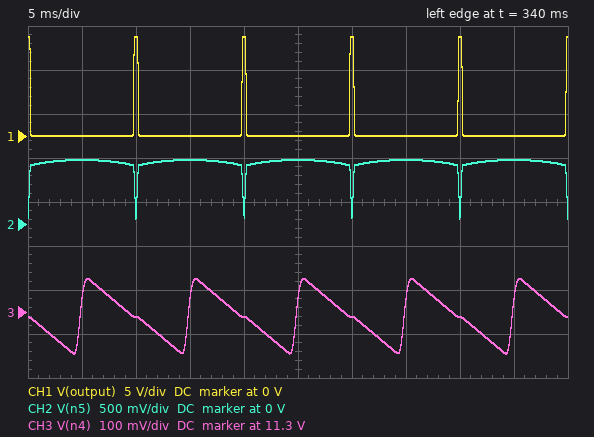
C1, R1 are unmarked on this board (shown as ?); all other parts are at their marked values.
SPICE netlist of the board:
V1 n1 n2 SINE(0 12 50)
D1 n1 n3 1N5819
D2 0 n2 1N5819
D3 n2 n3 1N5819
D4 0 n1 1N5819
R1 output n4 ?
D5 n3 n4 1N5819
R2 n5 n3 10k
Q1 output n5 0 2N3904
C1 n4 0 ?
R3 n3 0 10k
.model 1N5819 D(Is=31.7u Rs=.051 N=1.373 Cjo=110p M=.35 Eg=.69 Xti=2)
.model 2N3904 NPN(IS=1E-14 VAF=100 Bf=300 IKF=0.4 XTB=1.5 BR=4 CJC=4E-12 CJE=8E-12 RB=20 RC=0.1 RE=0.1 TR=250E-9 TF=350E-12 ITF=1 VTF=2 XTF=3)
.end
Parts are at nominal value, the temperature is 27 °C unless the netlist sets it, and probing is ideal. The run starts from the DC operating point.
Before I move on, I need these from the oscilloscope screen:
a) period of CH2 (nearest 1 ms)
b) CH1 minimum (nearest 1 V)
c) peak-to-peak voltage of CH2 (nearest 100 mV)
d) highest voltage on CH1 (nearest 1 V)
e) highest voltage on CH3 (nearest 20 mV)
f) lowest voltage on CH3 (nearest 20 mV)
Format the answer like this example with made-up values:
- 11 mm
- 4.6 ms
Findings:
- 10 ms
- 0 V
- 700 mV
- 11 V
- 11.38 V
- 11.20 V
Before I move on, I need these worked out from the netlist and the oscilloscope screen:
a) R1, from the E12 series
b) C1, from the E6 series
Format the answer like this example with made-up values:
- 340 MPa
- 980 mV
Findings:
- 8.2 kΩ
- 68 µF
